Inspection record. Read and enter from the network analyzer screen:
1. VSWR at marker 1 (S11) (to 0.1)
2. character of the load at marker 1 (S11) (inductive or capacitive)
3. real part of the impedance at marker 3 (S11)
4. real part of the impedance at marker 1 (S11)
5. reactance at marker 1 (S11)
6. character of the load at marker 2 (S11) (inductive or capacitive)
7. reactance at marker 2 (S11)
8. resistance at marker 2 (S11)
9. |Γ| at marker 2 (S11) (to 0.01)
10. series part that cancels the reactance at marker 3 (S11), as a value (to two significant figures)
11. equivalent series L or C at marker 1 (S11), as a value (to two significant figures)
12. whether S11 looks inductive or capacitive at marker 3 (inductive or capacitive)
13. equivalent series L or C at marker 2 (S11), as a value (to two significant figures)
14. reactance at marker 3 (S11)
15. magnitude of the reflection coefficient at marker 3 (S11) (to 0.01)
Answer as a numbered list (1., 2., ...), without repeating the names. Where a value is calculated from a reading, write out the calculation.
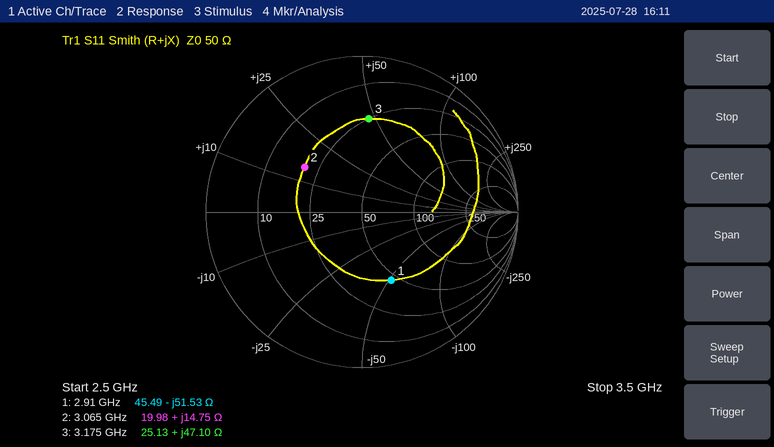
1. 2.8
2. capacitive
3. 25.13 Ω
4. 45.49 Ω
5. -51.53 Ω
6. inductive
7. +14.75 Ω
8. 19.98 Ω
9. 0.47
10. C = 1/(2π × 3.175 GHz × 47.1 Ω) ≈ 1.1 pF
11. C = 1/(2π × 2.91 GHz × 51.53 Ω) ≈ 1.1 pF
12. inductive
13. L = 14.75 Ω/(2π × 3.065 GHz) ≈ 766 pH, so 770 pH to two significant figures
14. +47.10 Ω
15. 0.60
